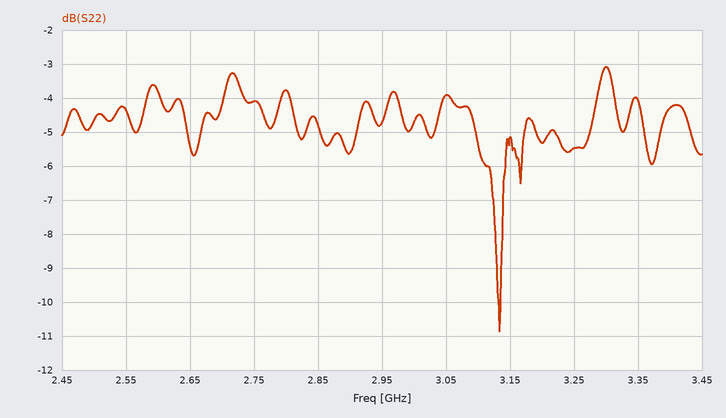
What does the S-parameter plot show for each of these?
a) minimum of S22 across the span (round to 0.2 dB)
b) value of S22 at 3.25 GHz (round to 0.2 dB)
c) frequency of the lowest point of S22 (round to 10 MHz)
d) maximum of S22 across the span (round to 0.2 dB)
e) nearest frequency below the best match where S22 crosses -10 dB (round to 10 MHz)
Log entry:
-10.8 dB
-5.4 dB
3.13 GHz
-3.0 dB
3.13 GHz
